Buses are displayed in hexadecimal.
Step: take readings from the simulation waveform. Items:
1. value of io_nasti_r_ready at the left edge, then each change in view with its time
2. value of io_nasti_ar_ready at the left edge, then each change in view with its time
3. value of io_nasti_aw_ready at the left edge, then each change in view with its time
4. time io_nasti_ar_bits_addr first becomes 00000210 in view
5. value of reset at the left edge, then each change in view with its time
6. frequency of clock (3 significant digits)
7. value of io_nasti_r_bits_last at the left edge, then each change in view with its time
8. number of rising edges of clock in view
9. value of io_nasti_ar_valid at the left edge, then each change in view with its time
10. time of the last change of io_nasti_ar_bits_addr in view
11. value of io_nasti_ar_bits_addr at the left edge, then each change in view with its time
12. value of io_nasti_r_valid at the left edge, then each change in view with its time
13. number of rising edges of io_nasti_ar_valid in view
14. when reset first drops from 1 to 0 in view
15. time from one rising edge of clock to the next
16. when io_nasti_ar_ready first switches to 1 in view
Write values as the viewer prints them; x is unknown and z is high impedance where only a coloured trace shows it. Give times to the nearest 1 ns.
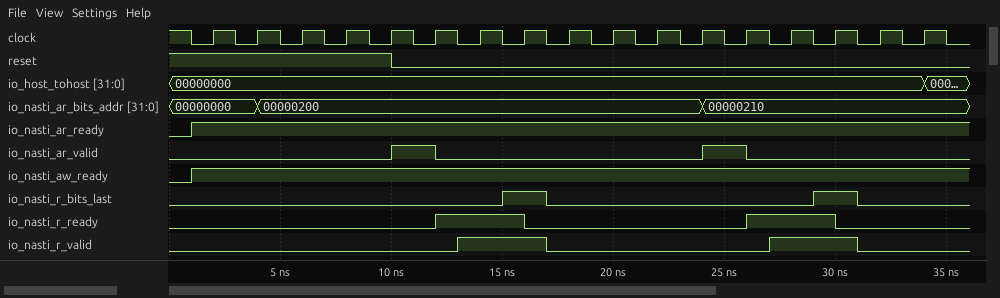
0, 1 at 12 ns, 0 at 16 ns, 1 at 26 ns, 0 at 30 ns
0, 1 at 1 ns
0, 1 at 1 ns
24 ns
1, 0 at 10 ns
500 MHz
0, 1 at 15 ns, 0 at 17 ns, 1 at 29 ns, 0 at 31 ns
17
0, 1 at 10 ns, 0 at 12 ns, 1 at 24 ns, 0 at 26 ns
24 ns
00000000, 00000200 at 4 ns, 00000210 at 24 ns
0, 1 at 13 ns, 0 at 17 ns, 1 at 27 ns, 0 at 31 ns
2
10 ns
2 ns
1 ns
